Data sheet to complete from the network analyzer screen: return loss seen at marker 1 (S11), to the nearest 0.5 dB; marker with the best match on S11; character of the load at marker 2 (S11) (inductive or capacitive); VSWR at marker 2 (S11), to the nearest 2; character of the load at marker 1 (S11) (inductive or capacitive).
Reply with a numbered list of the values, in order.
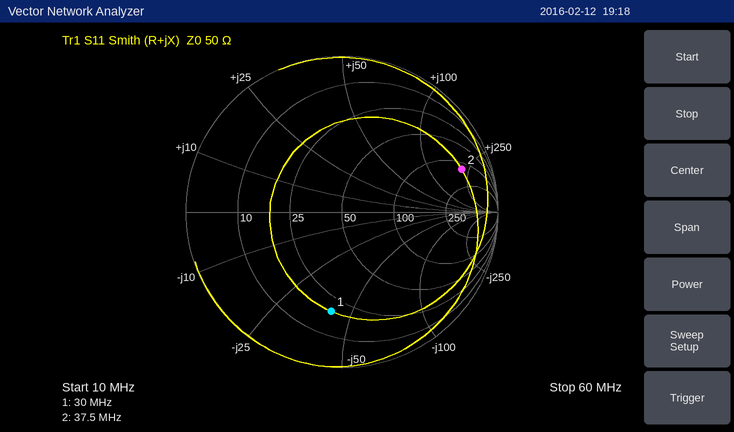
1. 4.0 dB
2. marker 1
3. inductive
4. 10
5. capacitive
